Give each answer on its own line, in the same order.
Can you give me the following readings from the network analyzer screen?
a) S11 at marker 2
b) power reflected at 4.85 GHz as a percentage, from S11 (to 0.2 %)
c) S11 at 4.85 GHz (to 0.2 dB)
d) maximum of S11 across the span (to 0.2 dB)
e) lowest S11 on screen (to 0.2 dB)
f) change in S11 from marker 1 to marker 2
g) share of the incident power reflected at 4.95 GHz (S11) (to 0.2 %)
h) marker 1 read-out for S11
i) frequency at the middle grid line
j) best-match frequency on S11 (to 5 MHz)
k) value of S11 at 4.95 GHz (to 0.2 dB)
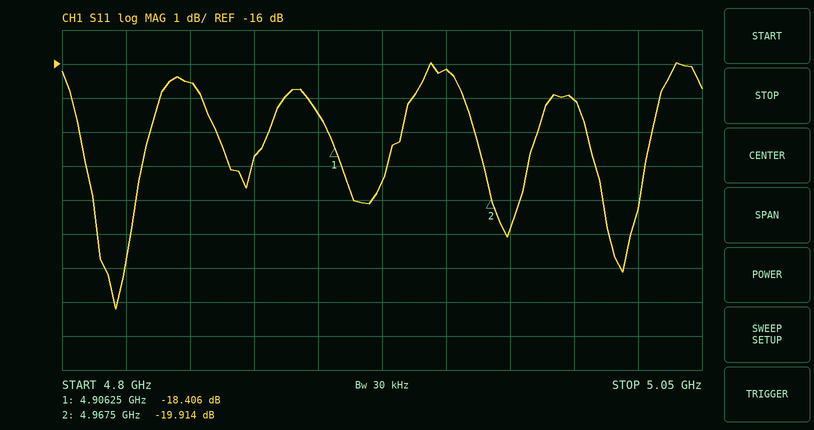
-19.914 dB
2.2 %
-16.6 dB
-16.0 dB
-23.2 dB
-1.508 dB
2.4 %
-18.406 dB
4.925 GHz
4.820 GHz
-16.2 dB
